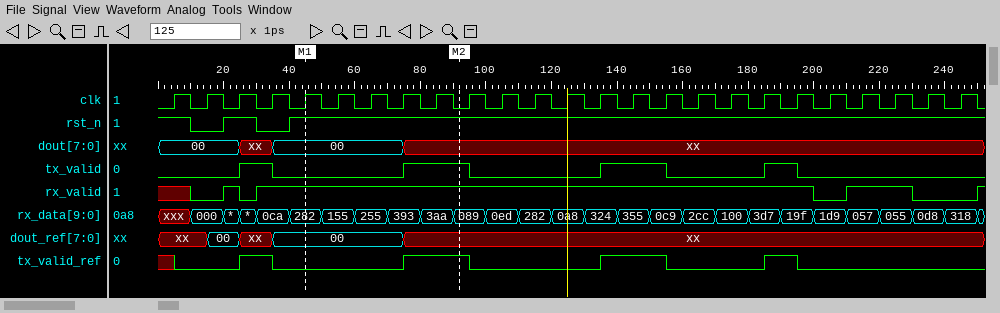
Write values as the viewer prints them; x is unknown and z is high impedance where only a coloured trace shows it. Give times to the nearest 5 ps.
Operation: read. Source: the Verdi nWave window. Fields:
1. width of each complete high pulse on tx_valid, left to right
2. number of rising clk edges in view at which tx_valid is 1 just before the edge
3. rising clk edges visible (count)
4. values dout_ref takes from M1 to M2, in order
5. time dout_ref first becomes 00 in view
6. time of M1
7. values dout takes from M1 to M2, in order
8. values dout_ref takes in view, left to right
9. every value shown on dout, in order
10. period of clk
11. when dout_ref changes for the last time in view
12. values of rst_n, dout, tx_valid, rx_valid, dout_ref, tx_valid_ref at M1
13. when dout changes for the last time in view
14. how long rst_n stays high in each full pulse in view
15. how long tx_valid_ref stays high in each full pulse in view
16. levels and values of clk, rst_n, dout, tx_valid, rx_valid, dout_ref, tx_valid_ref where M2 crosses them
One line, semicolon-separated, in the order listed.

10 ps, 20 ps, 20 ps, 10 ps; 6; 25; 00, xx; 15 ps; 45 ps; 00, xx; xx, 00, xx, 00, xx; 00, xx, 00, xx; 10 ps; 75 ps; rst_n=1, dout=00, tx_valid=0, rx_valid=1, dout_ref=00, tx_valid_ref=0; 75 ps; 10 ps; 10 ps, 20 ps, 20 ps, 10 ps; clk=0, rst_n=1, dout=xx, tx_valid=1, rx_valid=1, dout_ref=xx, tx_valid_ref=1
